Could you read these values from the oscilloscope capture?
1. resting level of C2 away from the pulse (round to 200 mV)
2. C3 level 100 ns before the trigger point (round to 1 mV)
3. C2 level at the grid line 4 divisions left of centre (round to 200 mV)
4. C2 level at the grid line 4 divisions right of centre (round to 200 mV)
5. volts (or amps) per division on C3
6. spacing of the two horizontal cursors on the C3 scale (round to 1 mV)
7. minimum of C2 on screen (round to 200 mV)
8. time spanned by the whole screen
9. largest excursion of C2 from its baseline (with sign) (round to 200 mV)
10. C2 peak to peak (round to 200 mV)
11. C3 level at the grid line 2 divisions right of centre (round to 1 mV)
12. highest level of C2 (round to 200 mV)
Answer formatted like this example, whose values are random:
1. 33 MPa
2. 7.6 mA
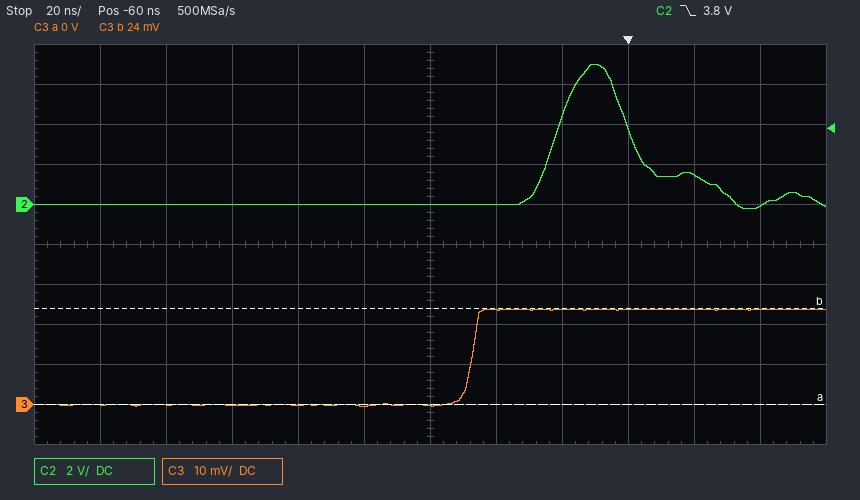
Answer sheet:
1. 0.0 V
2. 0 mV
3. 0.0 V
4. 1.4 V
5. 10 mV
6. 24 mV
7. -200 mV
8. 240 ns
9. +7.0 V
10. 7.2 V
11. 24 mV
12. 7.0 V
